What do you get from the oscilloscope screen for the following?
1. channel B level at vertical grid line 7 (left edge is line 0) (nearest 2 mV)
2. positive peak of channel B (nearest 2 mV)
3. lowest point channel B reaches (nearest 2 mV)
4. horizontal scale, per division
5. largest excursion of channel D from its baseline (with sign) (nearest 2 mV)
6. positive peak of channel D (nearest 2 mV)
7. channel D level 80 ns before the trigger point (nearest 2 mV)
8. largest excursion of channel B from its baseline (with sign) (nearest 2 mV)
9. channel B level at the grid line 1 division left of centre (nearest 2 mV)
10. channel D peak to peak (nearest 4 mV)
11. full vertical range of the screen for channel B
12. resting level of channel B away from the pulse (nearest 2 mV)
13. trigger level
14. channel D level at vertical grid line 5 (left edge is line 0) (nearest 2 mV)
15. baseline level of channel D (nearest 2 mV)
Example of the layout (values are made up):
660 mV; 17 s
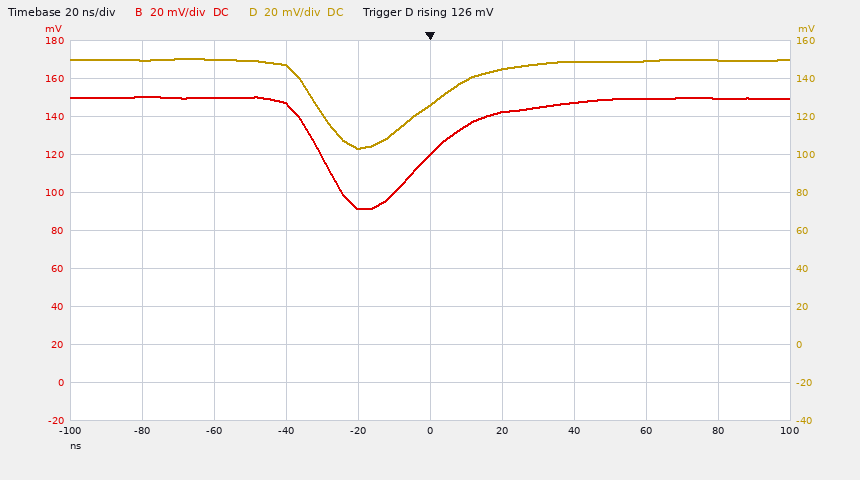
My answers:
148 mV; 150 mV; 92 mV; 20 ns; -46 mV; 150 mV; 150 mV; -58 mV; 92 mV; 48 mV; 200 mV; 150 mV; 126 mV; 126 mV; 150 mV
